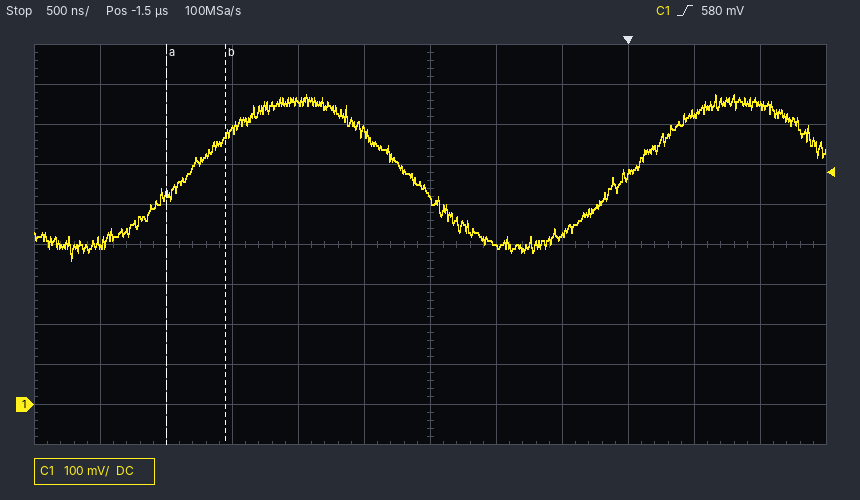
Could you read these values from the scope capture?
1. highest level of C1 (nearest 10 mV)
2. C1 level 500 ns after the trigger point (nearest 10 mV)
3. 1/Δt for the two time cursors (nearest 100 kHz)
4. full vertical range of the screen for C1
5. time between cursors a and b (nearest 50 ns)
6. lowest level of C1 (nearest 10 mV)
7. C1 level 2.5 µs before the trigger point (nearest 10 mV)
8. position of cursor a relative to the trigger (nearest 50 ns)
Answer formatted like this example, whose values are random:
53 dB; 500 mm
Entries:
780 mV; 730 mV; 2.2 MHz; 1 V; 450 ns; 360 mV; 760 mV; -3.50 µs
